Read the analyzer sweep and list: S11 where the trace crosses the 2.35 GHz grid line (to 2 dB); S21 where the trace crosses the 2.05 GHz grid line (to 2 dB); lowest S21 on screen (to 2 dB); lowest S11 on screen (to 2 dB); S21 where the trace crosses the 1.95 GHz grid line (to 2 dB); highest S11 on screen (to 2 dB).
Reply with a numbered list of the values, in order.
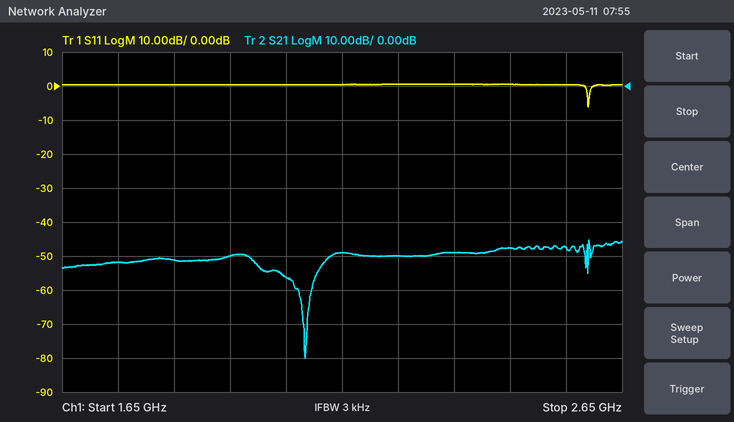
1. 0 dB
2. -56 dB
3. -80 dB
4. -6 dB
5. -50 dB
6. 0 dB
